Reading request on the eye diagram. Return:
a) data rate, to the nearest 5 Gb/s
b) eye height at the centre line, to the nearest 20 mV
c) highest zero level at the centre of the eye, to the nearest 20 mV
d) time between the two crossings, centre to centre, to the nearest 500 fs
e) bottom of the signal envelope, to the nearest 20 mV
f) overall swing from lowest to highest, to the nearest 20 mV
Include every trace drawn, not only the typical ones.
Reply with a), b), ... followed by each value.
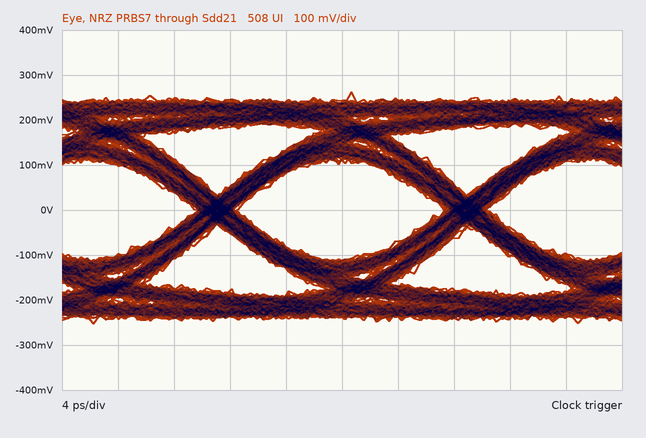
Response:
a) 55 Gb/s
b) 220 mV
c) -120 mV
d) 18.0 ps
e) -260 mV
f) 520 mV
